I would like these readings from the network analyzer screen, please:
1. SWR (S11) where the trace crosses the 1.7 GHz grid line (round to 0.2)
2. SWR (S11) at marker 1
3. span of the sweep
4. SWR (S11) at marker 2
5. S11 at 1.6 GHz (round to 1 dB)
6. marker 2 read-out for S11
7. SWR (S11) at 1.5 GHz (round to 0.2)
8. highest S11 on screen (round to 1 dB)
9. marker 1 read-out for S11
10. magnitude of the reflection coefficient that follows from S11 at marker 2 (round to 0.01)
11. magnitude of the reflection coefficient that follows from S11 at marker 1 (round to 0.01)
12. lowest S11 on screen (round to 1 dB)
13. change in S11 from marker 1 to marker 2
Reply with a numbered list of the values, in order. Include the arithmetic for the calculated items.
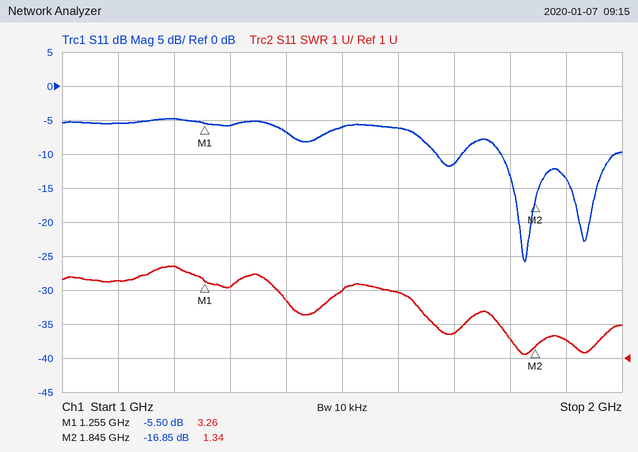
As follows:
1. 1.8
2. 3.26
3. 1 GHz
4. 1.34
5. -6 dB
6. -16.85 dB
7. 3.0
8. -5 dB
9. -5.50 dB
10. 10^(-16.85/20) ≈ 0.14
11. 10^(-5.5/20) ≈ 0.53
12. -26 dB
13. -16.85 − (-5.5) = -11.35 dB
